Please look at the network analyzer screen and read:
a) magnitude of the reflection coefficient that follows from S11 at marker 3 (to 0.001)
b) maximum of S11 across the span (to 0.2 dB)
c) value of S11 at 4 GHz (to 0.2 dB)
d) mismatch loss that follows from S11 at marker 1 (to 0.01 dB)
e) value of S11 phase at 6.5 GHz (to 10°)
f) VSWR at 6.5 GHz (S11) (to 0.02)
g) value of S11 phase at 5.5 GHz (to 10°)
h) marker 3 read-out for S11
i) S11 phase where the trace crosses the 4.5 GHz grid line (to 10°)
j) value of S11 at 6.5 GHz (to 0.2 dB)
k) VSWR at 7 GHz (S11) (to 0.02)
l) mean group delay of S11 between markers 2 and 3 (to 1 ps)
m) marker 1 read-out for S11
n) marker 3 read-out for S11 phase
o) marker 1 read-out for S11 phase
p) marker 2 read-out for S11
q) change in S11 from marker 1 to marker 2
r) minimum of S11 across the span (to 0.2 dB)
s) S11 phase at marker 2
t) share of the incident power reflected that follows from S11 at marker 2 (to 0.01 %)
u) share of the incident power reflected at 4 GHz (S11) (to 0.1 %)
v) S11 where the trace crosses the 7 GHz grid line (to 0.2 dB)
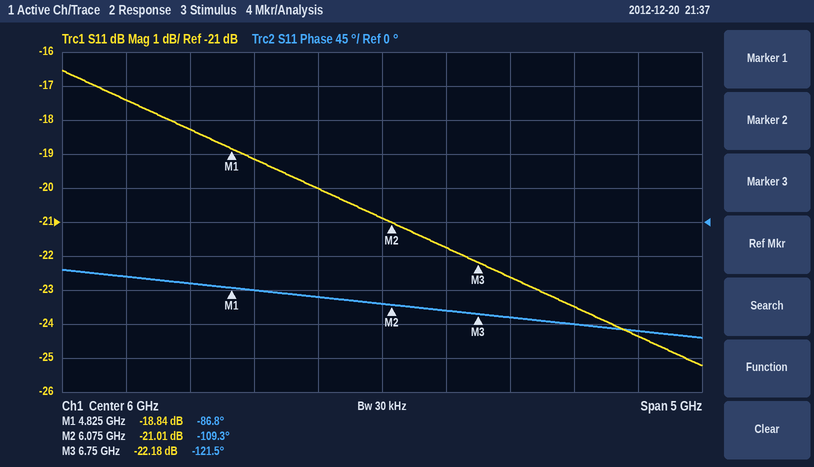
0.078
-16.6 dB
-17.4 dB
0.06 dB
-120°
1.18
-100°
-22.18 dB
-80°
-21.8 dB
1.16
50 ps
-18.84 dB
-121.5°
-86.8°
-21.01 dB
-2.17 dB
-25.2 dB
-109.3°
0.79 %
1.8 %
-22.6 dB
